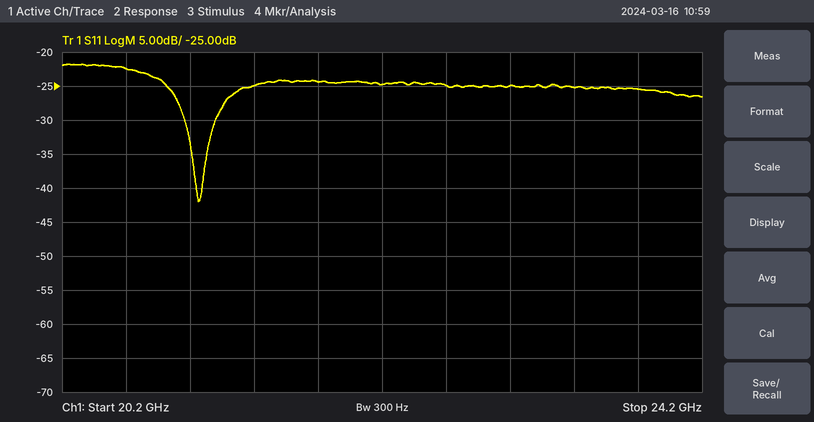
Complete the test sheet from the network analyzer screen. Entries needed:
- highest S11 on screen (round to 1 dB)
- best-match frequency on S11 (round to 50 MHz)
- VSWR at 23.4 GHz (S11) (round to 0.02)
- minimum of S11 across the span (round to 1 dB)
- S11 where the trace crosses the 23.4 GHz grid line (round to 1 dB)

-22 dB
21.05 GHz
1.12
-42 dB
-25 dB
